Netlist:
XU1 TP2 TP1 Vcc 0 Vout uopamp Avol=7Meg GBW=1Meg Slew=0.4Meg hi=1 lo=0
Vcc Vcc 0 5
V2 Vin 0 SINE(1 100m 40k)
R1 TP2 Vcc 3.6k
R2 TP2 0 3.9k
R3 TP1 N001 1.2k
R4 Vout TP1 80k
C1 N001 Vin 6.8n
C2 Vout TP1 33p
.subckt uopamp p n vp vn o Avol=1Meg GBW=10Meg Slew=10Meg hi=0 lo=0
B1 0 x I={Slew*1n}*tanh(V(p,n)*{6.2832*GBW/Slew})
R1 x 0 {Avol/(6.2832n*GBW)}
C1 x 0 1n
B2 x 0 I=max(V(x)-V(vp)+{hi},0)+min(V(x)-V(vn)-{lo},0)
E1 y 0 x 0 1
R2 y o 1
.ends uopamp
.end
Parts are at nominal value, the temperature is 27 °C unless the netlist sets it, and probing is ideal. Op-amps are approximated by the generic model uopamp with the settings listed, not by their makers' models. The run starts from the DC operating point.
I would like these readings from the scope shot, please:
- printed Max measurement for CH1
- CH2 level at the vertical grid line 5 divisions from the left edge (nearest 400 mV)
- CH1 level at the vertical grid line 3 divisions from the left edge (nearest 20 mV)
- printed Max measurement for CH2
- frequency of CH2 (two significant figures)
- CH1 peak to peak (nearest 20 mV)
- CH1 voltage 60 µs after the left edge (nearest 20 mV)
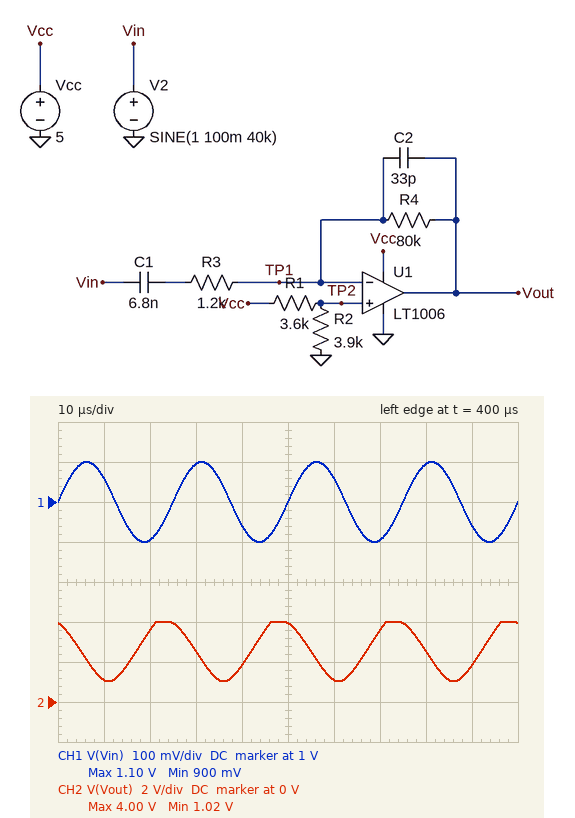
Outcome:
1.10 V
4.0 V
1.10 V
4.00 V
40 kHz
200 mV
1.06 V
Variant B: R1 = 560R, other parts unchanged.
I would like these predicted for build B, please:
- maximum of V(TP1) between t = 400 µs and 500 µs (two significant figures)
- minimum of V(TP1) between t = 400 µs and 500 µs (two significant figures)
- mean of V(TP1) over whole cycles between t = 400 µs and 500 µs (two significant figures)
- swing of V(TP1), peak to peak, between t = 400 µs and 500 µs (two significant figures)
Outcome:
4.1 V
3.9 V
4.0 V
200 mV
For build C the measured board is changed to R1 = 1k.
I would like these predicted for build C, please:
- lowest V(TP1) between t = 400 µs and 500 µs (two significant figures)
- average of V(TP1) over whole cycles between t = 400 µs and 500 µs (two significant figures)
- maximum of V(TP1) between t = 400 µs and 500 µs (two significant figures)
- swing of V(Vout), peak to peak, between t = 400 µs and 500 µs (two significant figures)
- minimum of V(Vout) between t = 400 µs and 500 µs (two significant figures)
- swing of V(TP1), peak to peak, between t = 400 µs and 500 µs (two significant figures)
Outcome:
3.8 V
3.9 V
4.0 V
460 mV
3.5 V
190 mV
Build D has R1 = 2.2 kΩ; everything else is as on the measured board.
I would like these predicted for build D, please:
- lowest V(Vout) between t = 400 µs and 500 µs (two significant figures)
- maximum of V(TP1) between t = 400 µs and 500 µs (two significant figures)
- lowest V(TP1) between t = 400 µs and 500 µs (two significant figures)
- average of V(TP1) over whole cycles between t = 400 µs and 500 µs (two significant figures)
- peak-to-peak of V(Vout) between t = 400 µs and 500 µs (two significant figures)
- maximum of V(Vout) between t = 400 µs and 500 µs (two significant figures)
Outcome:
1.9 V
3.3 V
3.1 V
3.2 V
2.1 V
4.0 V
